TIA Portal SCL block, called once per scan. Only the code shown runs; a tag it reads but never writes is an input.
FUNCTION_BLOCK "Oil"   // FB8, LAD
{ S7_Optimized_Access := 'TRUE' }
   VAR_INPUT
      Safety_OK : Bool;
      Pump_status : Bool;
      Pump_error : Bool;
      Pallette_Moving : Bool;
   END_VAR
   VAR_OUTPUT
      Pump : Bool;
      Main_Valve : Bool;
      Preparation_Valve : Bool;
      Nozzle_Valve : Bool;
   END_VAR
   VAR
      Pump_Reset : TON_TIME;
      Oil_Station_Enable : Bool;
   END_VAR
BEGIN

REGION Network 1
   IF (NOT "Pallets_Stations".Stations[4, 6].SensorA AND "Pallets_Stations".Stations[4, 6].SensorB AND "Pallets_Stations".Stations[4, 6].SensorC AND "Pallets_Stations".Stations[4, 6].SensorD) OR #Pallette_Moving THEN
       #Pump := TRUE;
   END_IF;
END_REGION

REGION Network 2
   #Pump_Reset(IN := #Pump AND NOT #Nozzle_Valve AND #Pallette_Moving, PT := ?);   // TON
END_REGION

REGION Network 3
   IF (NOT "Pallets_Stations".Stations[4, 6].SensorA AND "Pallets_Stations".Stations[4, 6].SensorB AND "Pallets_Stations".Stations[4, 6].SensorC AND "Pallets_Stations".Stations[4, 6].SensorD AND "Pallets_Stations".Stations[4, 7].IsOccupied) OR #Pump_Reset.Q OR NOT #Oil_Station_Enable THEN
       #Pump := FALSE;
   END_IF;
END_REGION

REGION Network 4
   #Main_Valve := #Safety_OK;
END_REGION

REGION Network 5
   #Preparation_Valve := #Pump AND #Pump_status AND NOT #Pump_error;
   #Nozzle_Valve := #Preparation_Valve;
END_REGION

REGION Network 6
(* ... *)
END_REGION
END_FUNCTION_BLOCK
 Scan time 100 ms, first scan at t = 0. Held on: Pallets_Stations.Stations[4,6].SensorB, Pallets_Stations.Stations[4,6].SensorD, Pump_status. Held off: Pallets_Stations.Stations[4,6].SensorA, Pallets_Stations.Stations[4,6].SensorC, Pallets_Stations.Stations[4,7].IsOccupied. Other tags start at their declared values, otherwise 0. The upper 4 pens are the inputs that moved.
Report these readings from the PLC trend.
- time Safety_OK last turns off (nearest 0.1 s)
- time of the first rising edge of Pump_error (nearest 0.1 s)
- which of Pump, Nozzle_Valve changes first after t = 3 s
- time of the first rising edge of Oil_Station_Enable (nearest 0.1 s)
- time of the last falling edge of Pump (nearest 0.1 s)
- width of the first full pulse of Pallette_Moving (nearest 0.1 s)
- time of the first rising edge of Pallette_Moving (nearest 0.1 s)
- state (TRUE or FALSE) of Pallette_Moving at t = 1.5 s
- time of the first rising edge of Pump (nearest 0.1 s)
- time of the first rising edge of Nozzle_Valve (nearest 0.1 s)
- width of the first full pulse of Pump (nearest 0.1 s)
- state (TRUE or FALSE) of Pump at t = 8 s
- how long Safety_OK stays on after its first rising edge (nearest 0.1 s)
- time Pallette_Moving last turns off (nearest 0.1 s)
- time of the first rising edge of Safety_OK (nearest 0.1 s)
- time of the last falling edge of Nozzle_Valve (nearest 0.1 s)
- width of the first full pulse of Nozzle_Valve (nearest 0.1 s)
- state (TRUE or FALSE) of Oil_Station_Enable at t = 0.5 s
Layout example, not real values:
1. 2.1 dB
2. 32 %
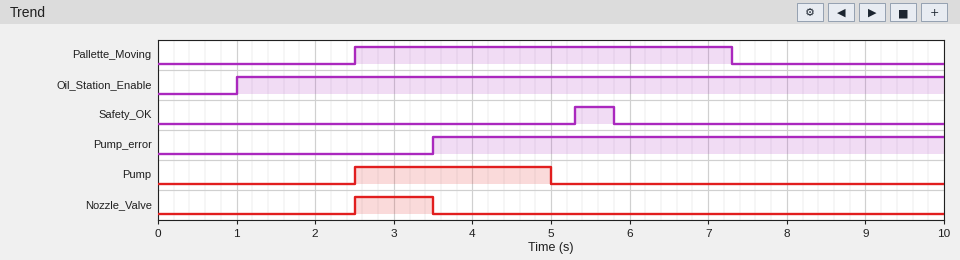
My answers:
1. 5.8 s
2. 3.5 s
3. Nozzle_Valve
4. 1.0 s
5. 5.0 s
6. 4.8 s
7. 2.5 s
8. FALSE
9. 2.5 s
10. 2.5 s
11. 2.5 s
12. FALSE
13. 0.5 s
14. 7.3 s
15. 5.3 s
16. 3.5 s
17. 1.0 s
18. FALSE
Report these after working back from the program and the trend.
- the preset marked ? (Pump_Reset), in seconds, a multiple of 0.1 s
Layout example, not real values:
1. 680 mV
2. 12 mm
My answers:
1. 1.4 s
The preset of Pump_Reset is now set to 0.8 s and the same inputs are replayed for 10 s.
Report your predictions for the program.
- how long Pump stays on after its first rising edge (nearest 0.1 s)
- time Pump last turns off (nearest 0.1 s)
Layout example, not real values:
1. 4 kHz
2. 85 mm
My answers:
1. 1.9 s
2. 4.4 s
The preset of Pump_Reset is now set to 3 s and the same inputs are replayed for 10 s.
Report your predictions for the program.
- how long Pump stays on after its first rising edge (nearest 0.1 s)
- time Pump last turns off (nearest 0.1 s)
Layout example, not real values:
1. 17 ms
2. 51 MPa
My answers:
1. 4.1 s
2. 6.6 s
